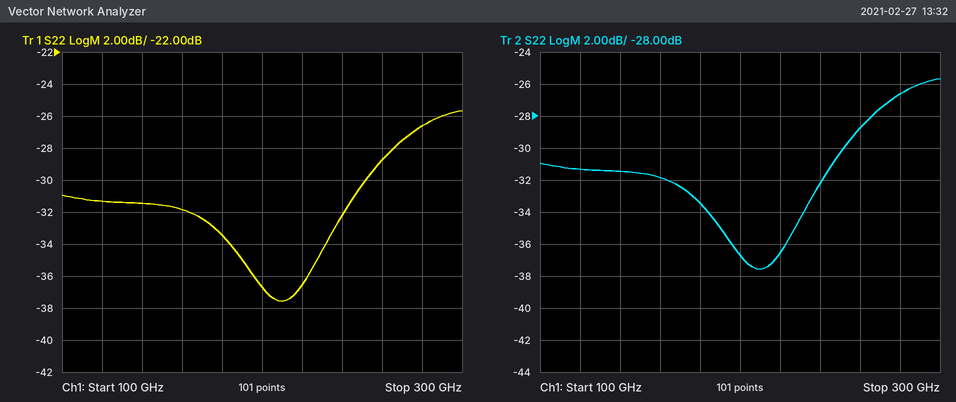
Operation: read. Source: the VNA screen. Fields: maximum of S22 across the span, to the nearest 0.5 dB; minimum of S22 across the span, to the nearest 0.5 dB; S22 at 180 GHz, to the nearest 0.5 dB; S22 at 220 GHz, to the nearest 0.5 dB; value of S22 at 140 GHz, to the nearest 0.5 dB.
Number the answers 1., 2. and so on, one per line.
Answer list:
1. -25.5 dB
2. -37.5 dB
3. -33.5 dB
4. -36.5 dB
5. -31.5 dB
